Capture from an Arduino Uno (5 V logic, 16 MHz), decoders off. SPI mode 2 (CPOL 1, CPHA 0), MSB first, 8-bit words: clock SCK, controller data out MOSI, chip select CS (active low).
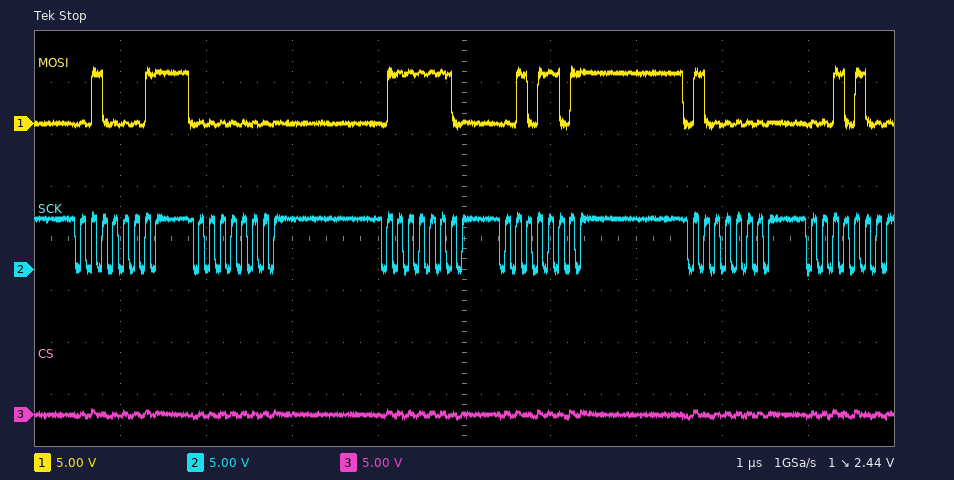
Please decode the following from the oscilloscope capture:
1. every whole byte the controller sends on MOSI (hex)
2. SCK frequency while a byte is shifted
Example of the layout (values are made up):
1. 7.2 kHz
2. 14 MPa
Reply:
1. 0x21 0x00 0x7E 0x2D 0x40 0x14
2. 8 MHz
